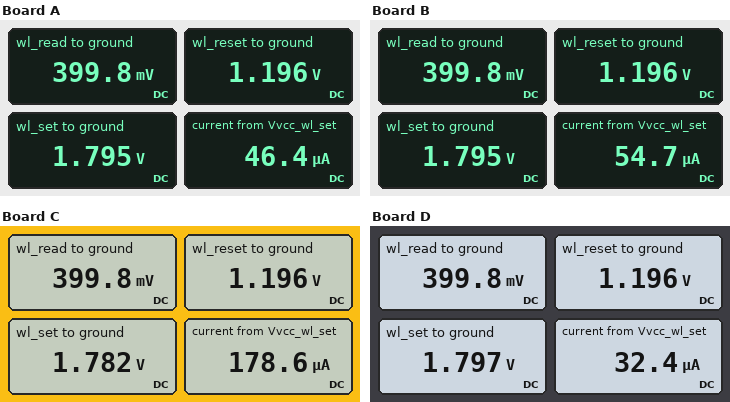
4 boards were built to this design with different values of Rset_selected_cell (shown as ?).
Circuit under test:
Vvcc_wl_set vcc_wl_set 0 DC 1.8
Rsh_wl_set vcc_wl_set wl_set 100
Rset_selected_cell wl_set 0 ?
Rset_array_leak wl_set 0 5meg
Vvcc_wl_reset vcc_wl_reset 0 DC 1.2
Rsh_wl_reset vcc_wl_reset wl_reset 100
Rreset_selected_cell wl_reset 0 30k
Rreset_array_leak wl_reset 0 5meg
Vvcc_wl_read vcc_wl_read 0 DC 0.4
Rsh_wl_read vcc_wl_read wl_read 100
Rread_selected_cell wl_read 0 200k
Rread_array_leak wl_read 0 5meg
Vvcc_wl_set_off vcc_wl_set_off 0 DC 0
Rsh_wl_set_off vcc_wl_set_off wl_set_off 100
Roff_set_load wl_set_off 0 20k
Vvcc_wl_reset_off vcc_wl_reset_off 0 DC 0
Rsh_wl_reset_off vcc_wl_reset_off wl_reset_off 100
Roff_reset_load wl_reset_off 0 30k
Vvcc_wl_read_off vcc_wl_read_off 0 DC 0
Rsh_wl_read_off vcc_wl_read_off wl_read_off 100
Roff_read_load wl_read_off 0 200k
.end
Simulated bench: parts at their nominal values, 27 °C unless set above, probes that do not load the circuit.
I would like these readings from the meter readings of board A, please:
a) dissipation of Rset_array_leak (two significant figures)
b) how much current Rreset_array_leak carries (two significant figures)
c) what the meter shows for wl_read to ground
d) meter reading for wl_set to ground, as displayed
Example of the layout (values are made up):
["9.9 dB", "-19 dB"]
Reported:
["640 nW", "240 nA", "399.8 mV", "1.795 V"]
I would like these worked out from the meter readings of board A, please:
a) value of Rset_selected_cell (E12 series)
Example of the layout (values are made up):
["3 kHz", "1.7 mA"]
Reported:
["39 kΩ"]
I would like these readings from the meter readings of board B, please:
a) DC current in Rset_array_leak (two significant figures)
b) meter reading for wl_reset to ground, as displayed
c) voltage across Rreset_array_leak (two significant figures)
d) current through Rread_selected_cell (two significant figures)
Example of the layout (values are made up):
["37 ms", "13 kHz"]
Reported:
["360 nA", "1.196 V", "1.2 V", "2.0 µA"]
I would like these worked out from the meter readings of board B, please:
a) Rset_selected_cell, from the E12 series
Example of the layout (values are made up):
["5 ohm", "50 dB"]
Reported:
["33 kΩ"]
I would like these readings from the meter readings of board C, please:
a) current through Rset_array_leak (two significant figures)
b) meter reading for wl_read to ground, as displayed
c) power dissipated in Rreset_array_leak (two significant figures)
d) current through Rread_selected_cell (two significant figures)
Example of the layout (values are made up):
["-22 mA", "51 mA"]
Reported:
["360 nA", "399.8 mV", "290 nW", "2.0 µA"]
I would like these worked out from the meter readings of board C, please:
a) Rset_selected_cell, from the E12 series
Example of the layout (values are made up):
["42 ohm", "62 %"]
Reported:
["10 kΩ"]
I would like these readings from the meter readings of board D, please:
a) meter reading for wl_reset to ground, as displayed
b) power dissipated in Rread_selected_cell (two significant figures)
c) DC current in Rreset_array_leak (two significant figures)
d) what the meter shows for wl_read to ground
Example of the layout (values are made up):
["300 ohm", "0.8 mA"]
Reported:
["1.196 V", "800 nW", "240 nA", "399.8 mV"]
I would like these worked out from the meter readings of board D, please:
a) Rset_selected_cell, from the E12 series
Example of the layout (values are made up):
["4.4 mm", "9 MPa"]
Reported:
["56 kΩ"]
